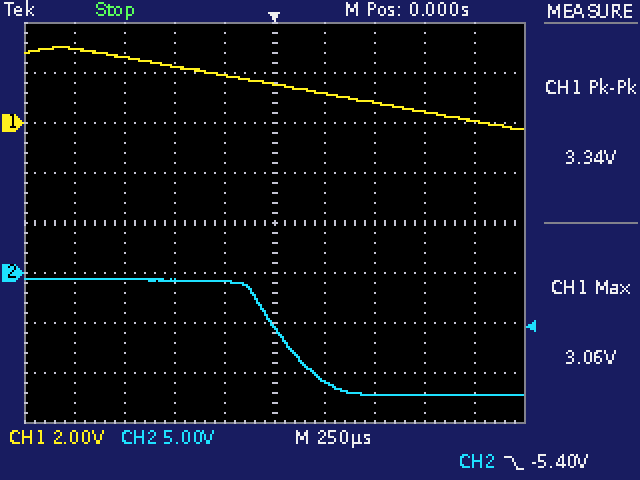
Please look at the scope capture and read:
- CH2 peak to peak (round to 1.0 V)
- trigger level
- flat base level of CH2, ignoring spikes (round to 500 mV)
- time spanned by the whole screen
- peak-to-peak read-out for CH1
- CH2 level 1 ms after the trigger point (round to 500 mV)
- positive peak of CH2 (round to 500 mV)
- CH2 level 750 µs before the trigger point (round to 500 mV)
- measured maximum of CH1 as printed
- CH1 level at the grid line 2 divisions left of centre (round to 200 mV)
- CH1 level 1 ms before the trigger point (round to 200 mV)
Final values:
12.0 V
-5.40 V
-12.0 V
2.5 ms
3.34 V
-12.0 V
-500 mV
-500 mV
3.06 V
2.2 V
3.0 V
